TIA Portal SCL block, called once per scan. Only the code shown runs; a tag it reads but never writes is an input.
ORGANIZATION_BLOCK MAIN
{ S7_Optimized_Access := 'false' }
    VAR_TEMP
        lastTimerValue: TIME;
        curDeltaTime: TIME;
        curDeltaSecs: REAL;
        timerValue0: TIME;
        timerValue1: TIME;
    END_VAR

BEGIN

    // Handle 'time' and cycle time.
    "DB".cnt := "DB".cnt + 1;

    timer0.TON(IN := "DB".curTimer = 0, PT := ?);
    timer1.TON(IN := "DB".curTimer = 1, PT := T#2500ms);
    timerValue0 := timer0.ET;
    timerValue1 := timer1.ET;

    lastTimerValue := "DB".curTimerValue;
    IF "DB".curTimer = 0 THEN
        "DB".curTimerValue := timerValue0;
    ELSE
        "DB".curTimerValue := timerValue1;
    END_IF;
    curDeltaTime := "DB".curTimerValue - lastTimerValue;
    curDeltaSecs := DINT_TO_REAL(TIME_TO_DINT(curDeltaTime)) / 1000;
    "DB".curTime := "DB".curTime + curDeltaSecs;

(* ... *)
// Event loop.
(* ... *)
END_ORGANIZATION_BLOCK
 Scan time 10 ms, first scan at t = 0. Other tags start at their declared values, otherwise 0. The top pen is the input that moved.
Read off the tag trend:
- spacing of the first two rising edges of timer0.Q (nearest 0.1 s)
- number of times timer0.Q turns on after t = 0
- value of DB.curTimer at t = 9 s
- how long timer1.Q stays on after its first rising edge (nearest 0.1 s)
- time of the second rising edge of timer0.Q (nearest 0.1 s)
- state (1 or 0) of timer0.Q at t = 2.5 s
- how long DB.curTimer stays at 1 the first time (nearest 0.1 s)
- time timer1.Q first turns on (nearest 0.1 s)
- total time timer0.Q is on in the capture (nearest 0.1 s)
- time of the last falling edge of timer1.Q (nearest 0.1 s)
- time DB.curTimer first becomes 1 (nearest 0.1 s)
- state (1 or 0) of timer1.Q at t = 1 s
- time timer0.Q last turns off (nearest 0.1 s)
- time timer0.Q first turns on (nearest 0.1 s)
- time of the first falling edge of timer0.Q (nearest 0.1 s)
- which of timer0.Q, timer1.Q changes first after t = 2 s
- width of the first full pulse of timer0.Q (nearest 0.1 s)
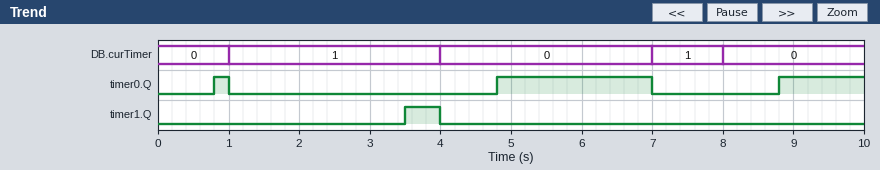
4.0 s
3
0
0.5 s
4.8 s
0
3.0 s
3.5 s
3.6 s
4.0 s
1.0 s
0
7.0 s
0.8 s
1.0 s
timer1.Q
0.2 s
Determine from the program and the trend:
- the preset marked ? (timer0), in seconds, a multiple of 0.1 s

0.8 s
